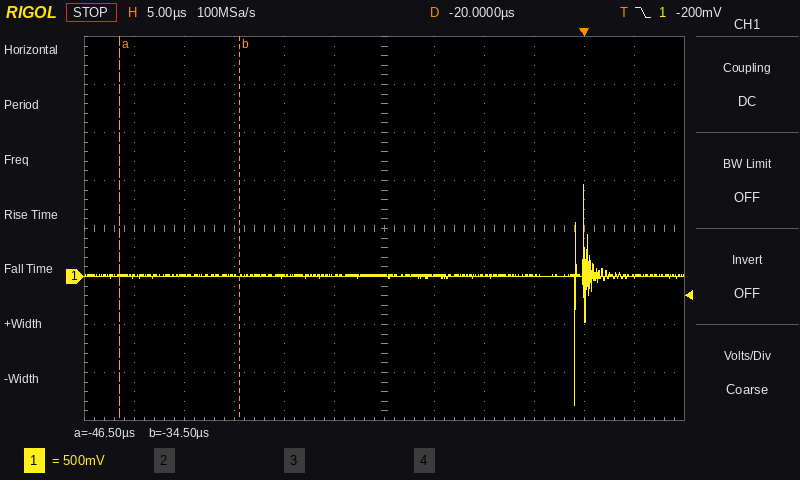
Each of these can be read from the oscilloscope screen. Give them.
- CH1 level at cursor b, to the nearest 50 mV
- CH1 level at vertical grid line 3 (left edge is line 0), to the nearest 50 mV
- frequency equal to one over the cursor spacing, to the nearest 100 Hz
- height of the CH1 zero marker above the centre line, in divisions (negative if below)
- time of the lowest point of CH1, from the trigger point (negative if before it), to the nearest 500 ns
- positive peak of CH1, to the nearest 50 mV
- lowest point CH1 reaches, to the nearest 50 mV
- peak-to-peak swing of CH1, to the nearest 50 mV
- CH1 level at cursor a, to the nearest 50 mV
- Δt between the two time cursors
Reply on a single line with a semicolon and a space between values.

0 mV; 0 mV; 83.3 kHz; -1.0 div; -1.0 µs; 950 mV; -1.35 V; 2.30 V; 0 mV; 12.0 µs
